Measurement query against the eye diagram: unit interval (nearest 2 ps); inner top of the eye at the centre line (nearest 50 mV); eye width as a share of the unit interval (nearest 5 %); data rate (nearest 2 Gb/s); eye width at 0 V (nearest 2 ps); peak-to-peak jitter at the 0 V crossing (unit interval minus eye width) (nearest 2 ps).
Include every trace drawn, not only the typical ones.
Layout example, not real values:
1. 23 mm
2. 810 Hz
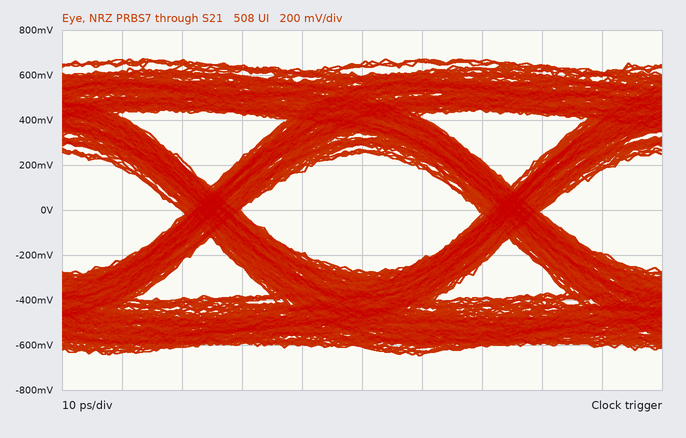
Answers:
1. 50 ps
2. 250 mV
3. 80 %
4. 20 Gb/s
5. 40 ps
6. 10 ps
